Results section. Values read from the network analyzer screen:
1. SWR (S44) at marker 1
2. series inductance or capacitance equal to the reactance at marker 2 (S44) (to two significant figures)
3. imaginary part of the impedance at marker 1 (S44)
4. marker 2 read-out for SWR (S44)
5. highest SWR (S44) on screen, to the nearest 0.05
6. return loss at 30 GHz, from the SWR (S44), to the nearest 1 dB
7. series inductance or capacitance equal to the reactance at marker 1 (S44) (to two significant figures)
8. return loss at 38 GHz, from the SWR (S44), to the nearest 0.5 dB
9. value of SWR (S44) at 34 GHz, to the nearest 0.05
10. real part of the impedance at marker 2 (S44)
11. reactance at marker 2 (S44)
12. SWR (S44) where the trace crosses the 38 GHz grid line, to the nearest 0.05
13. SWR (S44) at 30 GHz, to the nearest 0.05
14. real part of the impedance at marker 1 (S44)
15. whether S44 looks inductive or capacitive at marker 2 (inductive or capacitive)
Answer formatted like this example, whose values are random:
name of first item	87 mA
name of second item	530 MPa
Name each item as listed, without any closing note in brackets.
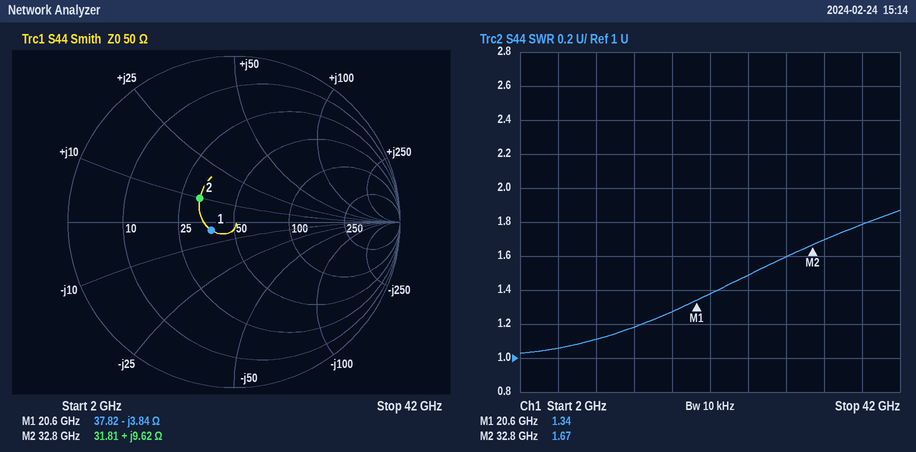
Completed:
SWR (S44) at marker 1	1.34
series inductance or capacitance equal to the reactance at marker 2 (S44)	47 pH
imaginary part of the impedance at marker 1	-3.84 Ω
marker 2 read-out for SWR	1.67
highest SWR (S44) on screen, to the nearest 0.05	1.85
return loss at 30 GHz, from the SWR (S44), to the nearest 1 dB	13 dB
series inductance or capacitance equal to the reactance at marker 1 (S44)	2.0 pF
return loss at 38 GHz, from the SWR (S44), to the nearest 0.5 dB	11.0 dB
value of SWR (S44) at 34 GHz, to the nearest 0.05	1.70
real part of the impedance at marker 2	31.81 Ω
reactance at marker 2	+9.62 Ω
SWR (S44) where the trace crosses the 38 GHz grid line, to the nearest 0.05	1.80
SWR (S44) at 30 GHz, to the nearest 0.05	1.60
real part of the impedance at marker 1	37.82 Ω
whether S44 looks inductive or capacitive at marker 2	inductive
